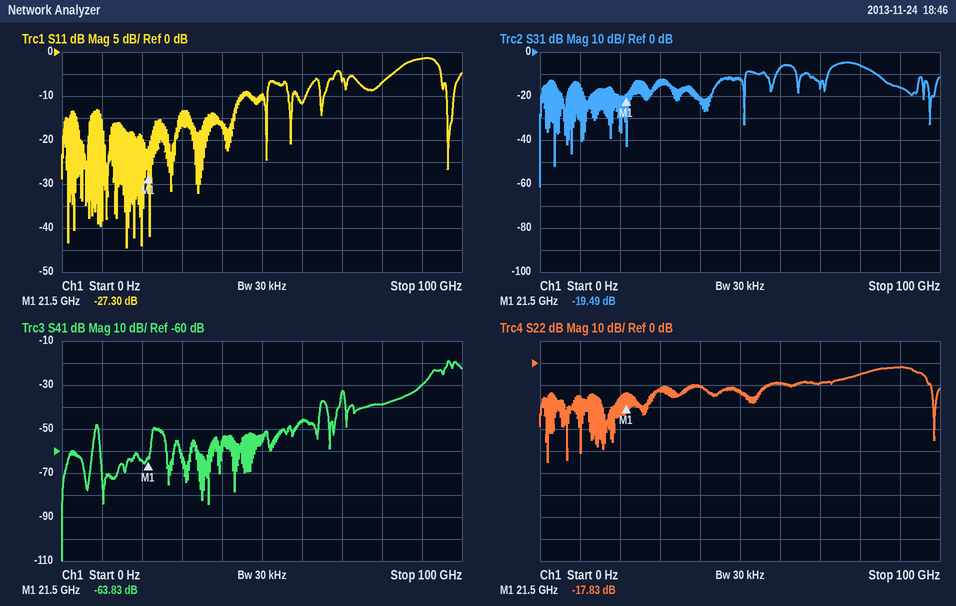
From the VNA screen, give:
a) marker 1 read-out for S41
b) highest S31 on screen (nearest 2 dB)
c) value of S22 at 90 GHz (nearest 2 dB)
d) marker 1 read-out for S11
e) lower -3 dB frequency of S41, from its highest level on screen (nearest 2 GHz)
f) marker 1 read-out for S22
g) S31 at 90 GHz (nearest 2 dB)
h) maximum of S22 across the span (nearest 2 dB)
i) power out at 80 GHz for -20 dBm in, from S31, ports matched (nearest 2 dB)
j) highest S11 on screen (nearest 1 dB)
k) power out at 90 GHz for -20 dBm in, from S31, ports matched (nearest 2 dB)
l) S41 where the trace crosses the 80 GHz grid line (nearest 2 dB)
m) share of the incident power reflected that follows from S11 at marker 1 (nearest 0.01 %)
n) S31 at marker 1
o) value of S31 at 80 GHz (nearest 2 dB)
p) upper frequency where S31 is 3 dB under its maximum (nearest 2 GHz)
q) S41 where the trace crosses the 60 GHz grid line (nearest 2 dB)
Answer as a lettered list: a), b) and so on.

a) -63.83 dB
b) -4 dB
c) -2 dB
d) -27.30 dB
e) 96 GHz
f) -17.83 dB
g) -16 dB
h) -2 dB
i) -26 dBm
j) -1 dB
k) -36 dBm
l) -38 dB
m) 0.19 %
n) -19.49 dB
o) -6 dB
p) 82 GHz
q) -46 dB
